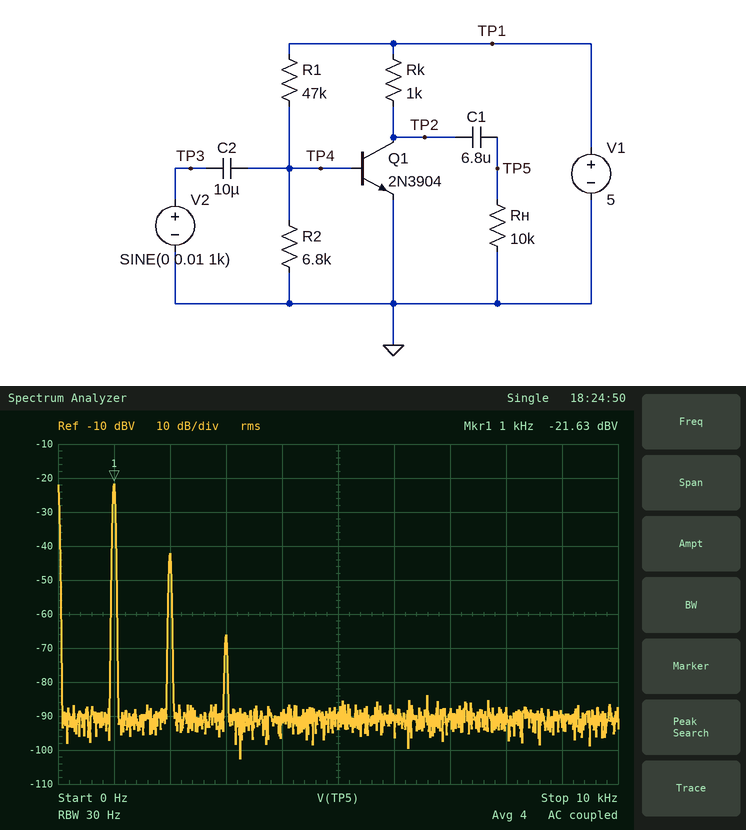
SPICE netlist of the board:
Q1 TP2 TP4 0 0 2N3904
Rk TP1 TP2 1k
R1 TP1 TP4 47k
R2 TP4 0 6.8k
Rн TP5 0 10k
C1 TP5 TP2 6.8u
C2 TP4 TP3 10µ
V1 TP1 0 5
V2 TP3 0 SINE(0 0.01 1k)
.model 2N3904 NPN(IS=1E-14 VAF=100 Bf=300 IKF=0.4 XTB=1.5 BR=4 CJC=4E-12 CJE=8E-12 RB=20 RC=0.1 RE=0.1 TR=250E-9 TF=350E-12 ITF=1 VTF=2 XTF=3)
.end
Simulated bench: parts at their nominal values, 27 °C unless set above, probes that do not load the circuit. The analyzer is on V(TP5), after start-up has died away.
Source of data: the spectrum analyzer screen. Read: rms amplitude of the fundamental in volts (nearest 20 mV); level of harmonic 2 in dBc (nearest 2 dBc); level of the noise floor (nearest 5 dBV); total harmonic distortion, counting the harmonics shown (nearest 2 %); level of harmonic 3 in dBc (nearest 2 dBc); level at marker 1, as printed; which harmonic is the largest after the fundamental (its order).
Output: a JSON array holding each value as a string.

["80 mV", "-20 dBc", "-90 dBV", "10 %", "-44 dBc", "-21.63 dBV", "2"]
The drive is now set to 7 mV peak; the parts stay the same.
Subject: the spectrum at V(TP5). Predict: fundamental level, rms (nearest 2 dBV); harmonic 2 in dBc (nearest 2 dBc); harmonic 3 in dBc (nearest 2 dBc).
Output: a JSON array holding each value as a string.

["-24 dBV", "-24 dBc", "-50 dBc"]
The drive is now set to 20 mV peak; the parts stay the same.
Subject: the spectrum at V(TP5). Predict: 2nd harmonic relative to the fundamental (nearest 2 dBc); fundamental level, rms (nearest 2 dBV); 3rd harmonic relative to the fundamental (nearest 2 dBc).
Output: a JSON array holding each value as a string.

["-14 dBc", "-16 dBV", "-32 dBc"]
